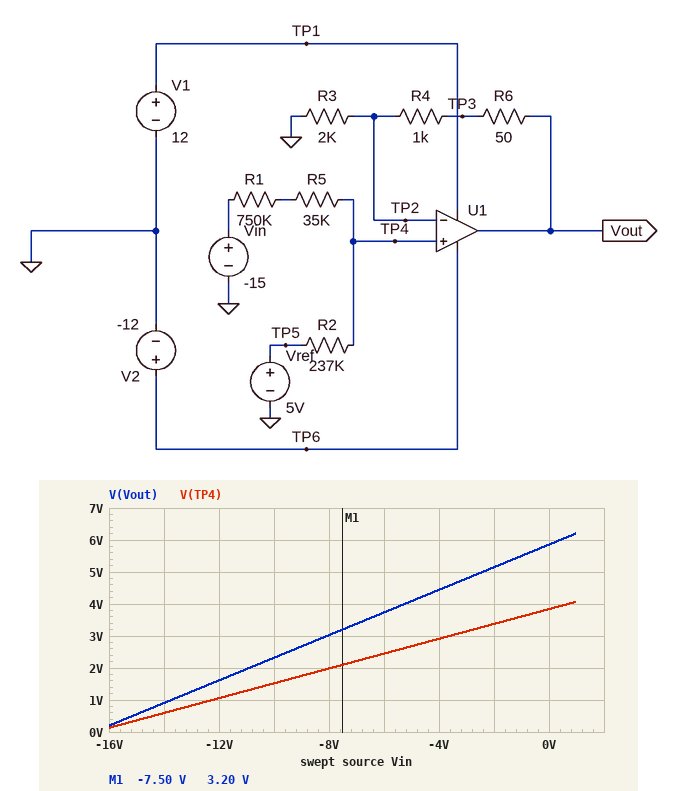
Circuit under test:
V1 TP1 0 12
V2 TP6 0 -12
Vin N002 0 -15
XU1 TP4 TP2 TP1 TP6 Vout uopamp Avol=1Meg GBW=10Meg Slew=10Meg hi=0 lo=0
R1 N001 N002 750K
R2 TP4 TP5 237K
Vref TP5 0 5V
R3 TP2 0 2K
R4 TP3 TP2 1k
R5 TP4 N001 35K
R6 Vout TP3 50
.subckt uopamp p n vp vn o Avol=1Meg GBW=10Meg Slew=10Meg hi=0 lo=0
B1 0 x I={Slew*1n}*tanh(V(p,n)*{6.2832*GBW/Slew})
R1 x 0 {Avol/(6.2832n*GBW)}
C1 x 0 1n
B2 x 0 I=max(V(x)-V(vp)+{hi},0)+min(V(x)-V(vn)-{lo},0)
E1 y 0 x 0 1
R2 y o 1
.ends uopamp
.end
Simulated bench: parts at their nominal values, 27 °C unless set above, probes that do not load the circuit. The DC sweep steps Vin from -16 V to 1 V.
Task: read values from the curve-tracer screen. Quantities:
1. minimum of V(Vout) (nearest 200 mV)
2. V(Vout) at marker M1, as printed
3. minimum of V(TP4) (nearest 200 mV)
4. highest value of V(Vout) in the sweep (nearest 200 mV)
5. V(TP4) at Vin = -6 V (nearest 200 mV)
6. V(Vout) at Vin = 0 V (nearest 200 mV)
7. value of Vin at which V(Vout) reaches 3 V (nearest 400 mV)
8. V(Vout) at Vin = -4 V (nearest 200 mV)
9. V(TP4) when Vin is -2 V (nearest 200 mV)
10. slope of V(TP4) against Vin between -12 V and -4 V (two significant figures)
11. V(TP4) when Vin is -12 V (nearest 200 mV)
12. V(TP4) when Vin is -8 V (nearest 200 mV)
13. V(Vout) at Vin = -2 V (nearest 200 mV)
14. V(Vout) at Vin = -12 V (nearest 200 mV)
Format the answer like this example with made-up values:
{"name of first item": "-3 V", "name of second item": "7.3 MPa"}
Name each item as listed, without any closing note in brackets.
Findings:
{"minimum of V(Vout)": "200 mV", "V(Vout) at marker M1, as printed": "3.20 V", "minimum of V(TP4)": "200 mV", "highest value of V(Vout) in the sweep": "6.2 V", "V(TP4) at Vin = -6 V": "2.4 V", "V(Vout) at Vin = 0 V": "5.8 V", "value of Vin at which V(Vout) reaches 3 V": "-8.0 V", "V(Vout) at Vin = -4 V": "4.4 V", "V(TP4) when Vin is -2 V": "3.4 V", "slope of V(TP4) against Vin between -12 V and -4 V": "0.23 V/V", "V(TP4) when Vin is -12 V": "1.0 V", "V(TP4) when Vin is -8 V": "2.0 V", "V(Vout) at Vin = -2 V": "5.2 V", "V(Vout) at Vin = -12 V": "1.6 V"}
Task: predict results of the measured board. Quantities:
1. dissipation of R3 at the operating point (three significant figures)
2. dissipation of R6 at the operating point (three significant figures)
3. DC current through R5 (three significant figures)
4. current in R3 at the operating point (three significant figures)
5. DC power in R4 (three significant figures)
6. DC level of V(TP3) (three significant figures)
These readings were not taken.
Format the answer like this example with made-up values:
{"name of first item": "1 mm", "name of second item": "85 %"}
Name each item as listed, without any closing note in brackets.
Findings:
{"dissipation of R3 at the operating point": "65.5 µW", "dissipation of R6 at the operating point": "1.64 µW", "DC current through R5": "19.6 µA", "current in R3 at the operating point": "181 µA", "DC power in R4": "32.8 µW", "DC level of V(TP3)": "543 mV"}
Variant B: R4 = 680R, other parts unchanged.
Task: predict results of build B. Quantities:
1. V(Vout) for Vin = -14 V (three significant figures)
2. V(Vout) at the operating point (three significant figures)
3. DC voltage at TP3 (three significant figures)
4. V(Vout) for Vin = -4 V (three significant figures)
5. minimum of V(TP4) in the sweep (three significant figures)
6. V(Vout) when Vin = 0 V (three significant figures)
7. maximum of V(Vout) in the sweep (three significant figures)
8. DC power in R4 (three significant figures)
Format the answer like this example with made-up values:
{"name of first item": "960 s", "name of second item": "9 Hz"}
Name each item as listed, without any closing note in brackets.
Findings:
{"V(Vout) for Vin = -14 V": "811 mV", "V(Vout) at the operating point": "494 mV", "DC voltage at TP3": "485 mV", "V(Vout) for Vin = -4 V": "3.98 V", "minimum of V(TP4) in the sweep": "130 mV", "V(Vout) when Vin = 0 V": "5.24 V", "maximum of V(Vout) in the sweep": "5.56 V", "DC power in R4": "22.3 µW"}
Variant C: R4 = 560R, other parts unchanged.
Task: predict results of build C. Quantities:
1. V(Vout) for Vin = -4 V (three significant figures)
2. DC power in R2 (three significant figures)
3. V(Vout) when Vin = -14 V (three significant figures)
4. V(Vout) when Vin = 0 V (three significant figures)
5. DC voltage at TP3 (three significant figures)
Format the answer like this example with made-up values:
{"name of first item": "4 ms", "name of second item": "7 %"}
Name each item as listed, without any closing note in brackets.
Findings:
{"V(Vout) for Vin = -4 V": "3.80 V", "DC power in R2": "90.8 µW", "V(Vout) when Vin = -14 V": "775 mV", "V(Vout) when Vin = 0 V": "5.01 V", "DC voltage at TP3": "463 mV"}
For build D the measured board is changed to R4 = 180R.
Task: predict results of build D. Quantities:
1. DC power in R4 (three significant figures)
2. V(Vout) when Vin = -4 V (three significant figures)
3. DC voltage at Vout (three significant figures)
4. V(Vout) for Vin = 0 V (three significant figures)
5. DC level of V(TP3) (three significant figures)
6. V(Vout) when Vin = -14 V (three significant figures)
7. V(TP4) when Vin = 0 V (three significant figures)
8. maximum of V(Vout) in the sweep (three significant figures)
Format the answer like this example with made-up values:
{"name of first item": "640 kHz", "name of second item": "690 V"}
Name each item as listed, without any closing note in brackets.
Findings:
{"DC power in R4": "5.90 µW", "V(Vout) when Vin = -4 V": "3.25 V", "DC voltage at Vout": "404 mV", "V(Vout) for Vin = 0 V": "4.28 V", "DC level of V(TP3)": "395 mV", "V(Vout) when Vin = -14 V": "662 mV", "V(TP4) when Vin = 0 V": "3.84 V", "maximum of V(Vout) in the sweep": "4.54 V"}
